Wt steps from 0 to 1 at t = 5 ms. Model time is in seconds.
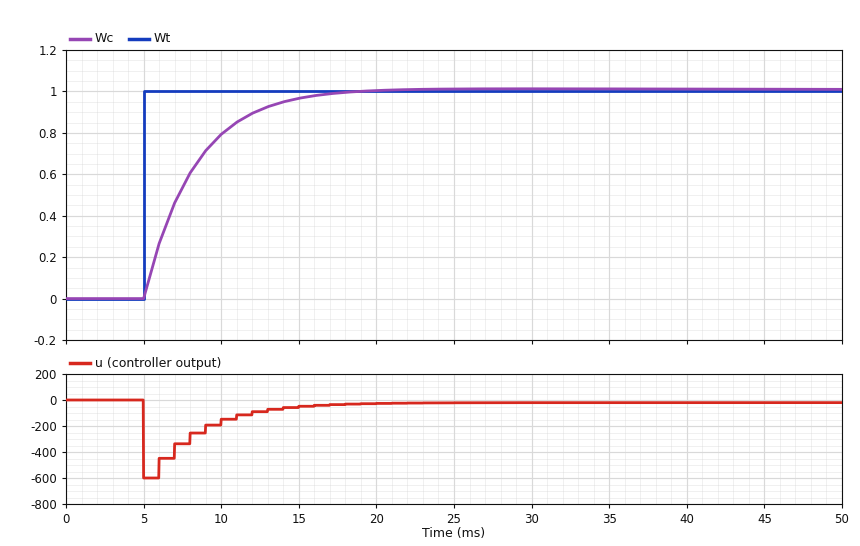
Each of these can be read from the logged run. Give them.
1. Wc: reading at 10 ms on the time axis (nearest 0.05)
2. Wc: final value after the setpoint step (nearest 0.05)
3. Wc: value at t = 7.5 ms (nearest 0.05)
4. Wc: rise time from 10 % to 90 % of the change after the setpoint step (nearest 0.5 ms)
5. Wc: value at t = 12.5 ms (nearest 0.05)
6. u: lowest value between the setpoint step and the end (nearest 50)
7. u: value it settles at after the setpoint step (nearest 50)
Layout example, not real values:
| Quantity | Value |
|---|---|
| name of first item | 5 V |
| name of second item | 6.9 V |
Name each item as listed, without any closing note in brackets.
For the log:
| Quantity | Value |
|---|---|
| Wc: reading at 10 ms on the time axis | 0.80 |
| Wc: final value after the setpoint step | 1.00 |
| Wc: value at t = 7.5 ms | 0.55 |
| Wc: rise time from 10 % to 90 % of the change after the setpoint step | 7.0 ms |
| Wc: value at t = 12.5 ms | 0.90 |
| u: lowest value between the setpoint step and the end | -600 |
| u: value it settles at after the setpoint step | 0 |
